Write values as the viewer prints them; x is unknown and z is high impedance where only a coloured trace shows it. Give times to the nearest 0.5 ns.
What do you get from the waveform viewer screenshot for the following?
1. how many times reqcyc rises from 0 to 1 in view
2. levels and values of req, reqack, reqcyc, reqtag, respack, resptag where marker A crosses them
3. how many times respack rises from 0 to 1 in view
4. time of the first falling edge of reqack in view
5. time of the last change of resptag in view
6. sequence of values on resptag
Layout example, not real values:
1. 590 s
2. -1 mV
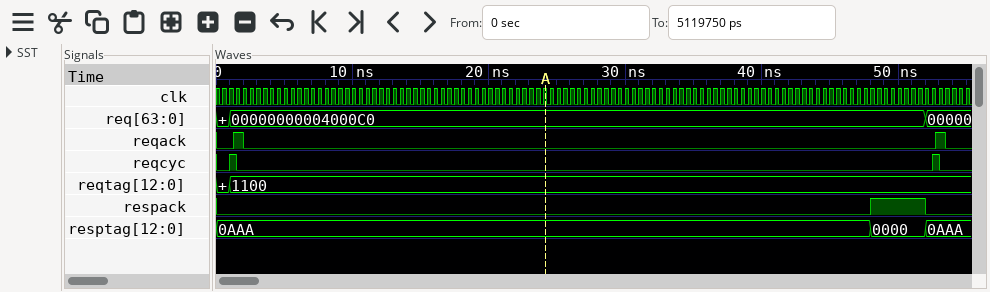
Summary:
1. 2
2. req=00000000004000C0, reqack=0, reqcyc=0, reqtag=1100, respack=0, resptag=0AAA
3. 1
4. 2 ns
5. 52 ns
6. 0AAA, 0000, 0AAA
